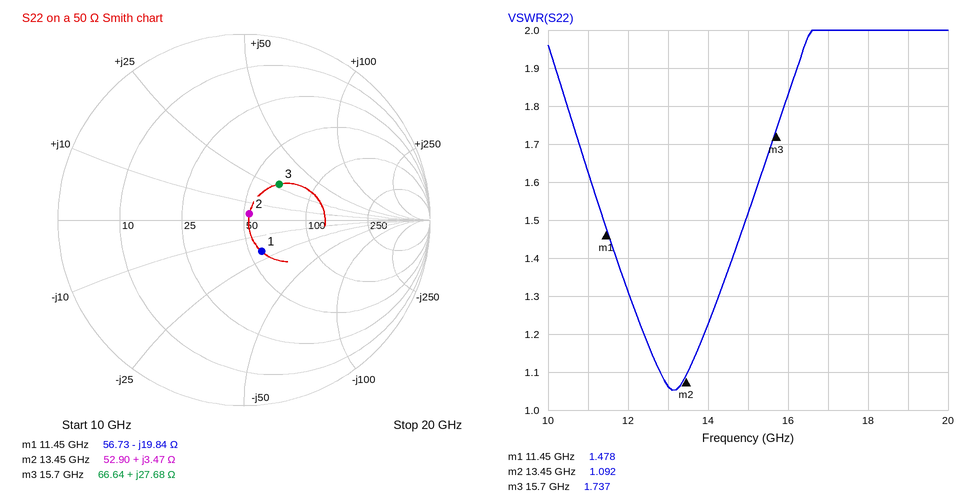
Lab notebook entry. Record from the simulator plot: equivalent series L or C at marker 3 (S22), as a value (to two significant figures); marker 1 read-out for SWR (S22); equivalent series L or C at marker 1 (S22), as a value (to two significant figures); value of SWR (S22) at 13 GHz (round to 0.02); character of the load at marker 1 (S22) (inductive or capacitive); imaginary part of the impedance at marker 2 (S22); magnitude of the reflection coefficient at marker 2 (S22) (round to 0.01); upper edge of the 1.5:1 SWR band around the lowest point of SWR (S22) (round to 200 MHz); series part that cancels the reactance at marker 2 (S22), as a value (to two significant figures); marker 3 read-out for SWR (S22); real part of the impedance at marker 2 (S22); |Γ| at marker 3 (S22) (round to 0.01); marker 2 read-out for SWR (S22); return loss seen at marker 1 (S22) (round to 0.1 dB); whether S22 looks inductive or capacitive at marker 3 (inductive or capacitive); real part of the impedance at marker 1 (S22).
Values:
280 pH
1.478
700 fF
1.06
capacitive
+3.47 Ω
0.04
15.0 GHz
3.4 pF
1.737
52.90 Ω
0.27
1.092
14.3 dB
inductive
56.73 Ω
